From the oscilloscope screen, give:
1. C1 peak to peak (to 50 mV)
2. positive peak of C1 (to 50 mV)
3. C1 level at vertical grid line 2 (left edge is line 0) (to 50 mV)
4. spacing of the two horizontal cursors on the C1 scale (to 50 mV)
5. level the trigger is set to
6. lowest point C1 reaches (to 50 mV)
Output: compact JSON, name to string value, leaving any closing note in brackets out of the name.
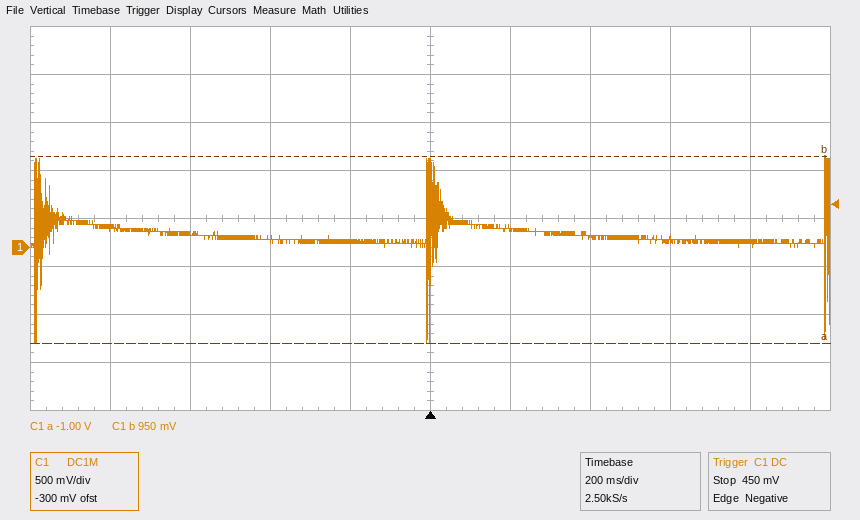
{"C1 peak to peak": "1.95 V", "positive peak of C1": "950 mV", "C1 level at vertical grid line 2 (left edge is line 0)": "150 mV", "spacing of the two horizontal cursors on the C1 scale": "1.95 V", "level the trigger is set to": "450 mV", "lowest point C1 reaches": "-1.00 V"}
